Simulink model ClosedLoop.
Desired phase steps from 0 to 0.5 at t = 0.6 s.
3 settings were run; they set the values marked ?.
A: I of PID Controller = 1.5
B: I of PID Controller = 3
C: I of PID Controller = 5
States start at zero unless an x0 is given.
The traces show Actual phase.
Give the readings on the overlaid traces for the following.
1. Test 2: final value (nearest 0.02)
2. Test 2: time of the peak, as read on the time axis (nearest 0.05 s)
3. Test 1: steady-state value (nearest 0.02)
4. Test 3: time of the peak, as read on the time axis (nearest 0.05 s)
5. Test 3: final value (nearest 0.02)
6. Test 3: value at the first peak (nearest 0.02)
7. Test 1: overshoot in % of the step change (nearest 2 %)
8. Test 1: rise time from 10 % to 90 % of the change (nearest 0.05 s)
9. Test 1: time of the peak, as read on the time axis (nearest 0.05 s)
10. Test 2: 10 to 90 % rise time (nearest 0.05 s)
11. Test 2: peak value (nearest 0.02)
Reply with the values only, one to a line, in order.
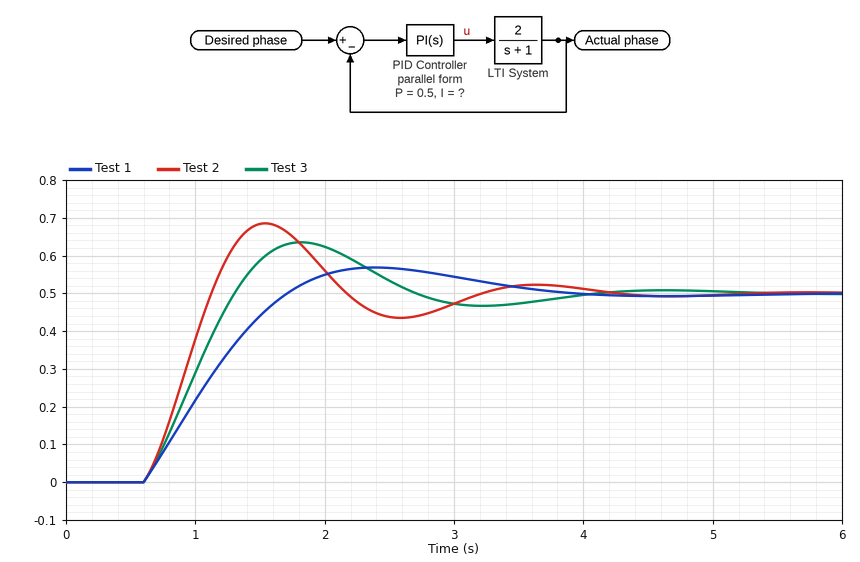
0.50
1.55 s
0.50
1.80 s
0.50
0.64
14 %
0.85 s
2.40 s
0.40 s
0.68
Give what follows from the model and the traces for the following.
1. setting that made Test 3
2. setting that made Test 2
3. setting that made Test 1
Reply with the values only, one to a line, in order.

B
C
A
